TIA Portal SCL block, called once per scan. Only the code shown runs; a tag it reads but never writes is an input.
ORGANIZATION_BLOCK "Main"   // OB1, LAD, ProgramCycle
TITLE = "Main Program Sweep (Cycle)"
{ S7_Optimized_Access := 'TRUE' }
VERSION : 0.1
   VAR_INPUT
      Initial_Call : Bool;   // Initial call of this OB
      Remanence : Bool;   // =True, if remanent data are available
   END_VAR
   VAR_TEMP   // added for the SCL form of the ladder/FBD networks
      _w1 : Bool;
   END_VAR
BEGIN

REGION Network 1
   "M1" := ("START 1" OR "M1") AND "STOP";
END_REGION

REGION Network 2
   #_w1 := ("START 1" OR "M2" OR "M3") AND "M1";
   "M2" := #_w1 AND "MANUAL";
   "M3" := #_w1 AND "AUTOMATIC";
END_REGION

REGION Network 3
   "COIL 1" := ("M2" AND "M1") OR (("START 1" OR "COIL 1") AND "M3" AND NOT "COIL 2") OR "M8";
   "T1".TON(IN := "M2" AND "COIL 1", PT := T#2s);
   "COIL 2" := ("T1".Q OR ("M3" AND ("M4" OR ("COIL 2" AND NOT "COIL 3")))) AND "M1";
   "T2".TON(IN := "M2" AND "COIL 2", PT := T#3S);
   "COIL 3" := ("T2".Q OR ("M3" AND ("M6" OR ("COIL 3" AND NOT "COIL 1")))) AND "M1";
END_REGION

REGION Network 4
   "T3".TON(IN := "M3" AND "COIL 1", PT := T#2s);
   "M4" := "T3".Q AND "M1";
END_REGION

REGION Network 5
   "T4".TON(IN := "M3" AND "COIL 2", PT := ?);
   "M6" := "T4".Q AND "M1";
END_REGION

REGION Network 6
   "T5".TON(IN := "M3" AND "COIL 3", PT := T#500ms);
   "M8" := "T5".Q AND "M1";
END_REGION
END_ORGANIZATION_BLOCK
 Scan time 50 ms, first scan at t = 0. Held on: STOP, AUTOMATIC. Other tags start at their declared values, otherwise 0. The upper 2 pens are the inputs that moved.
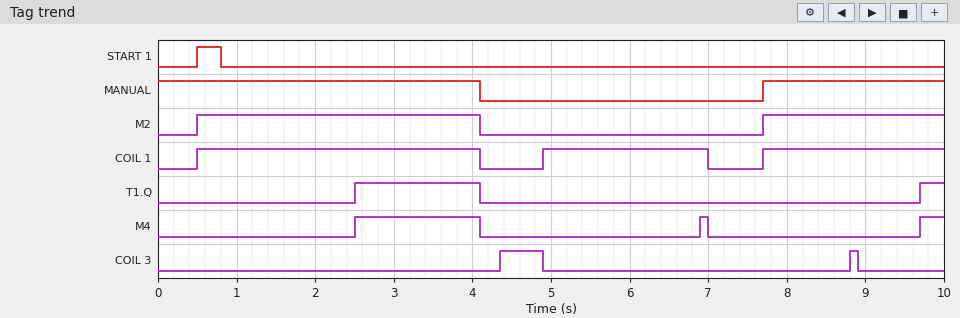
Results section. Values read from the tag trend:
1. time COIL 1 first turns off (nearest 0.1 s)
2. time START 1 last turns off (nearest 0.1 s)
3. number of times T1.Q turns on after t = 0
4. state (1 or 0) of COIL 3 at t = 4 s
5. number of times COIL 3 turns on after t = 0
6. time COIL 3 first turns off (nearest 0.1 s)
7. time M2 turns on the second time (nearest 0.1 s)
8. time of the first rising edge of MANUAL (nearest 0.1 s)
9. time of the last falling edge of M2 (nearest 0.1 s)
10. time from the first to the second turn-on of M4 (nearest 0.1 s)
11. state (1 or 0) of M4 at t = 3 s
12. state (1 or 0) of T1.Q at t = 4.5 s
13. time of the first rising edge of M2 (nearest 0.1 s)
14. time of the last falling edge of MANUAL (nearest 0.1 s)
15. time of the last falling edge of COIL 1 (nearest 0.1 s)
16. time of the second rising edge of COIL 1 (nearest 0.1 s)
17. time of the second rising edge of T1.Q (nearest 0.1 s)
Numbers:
4.1 s
0.8 s
2
0
2
4.9 s
7.7 s
7.7 s
4.1 s
4.4 s
1
0
0.5 s
4.1 s
7.0 s
4.9 s
9.7 s
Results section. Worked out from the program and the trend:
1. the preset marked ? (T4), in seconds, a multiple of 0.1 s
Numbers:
1.8 s
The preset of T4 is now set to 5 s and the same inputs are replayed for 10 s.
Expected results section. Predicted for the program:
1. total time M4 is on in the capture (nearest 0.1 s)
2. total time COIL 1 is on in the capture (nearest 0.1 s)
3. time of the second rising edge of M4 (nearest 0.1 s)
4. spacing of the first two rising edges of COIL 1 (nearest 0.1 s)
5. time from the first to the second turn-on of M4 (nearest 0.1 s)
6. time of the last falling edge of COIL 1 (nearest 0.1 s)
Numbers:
1.9 s
5.9 s
9.7 s
7.2 s
7.2 s
4.1 s
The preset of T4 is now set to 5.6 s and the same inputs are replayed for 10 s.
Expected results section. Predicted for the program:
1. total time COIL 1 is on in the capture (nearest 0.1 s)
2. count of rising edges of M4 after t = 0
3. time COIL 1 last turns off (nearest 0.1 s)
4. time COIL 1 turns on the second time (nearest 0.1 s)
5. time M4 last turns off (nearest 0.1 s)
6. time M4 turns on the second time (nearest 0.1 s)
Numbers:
5.9 s
2
4.1 s
7.7 s
4.1 s
9.7 s
